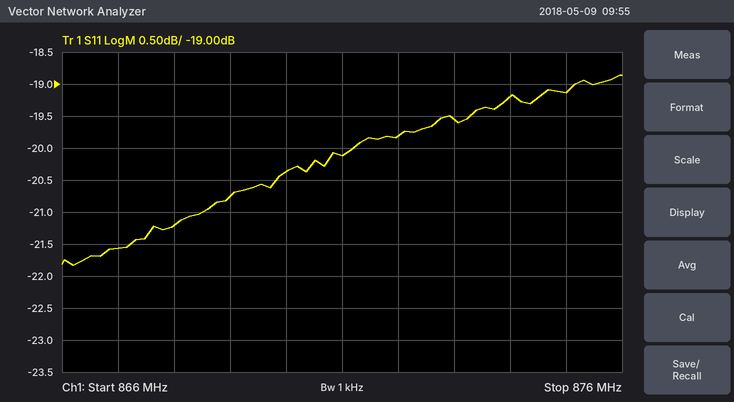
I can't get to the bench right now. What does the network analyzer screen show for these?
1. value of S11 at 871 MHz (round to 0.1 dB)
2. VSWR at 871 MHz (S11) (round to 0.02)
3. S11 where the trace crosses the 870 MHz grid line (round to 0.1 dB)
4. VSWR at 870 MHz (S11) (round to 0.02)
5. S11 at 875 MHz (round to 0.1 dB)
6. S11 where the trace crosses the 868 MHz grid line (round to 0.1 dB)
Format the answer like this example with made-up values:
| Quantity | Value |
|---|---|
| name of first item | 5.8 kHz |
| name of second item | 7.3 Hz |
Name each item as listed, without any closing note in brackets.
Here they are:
| Quantity | Value |
|---|---|
| value of S11 at 871 MHz | -20.1 dB |
| VSWR at 871 MHz (S11) | 1.22 |
| S11 where the trace crosses the 870 MHz grid line | -20.4 dB |
| VSWR at 870 MHz (S11) | 1.22 |
| S11 at 875 MHz | -19.1 dB |
| S11 where the trace crosses the 868 MHz grid line | -21.2 dB |
